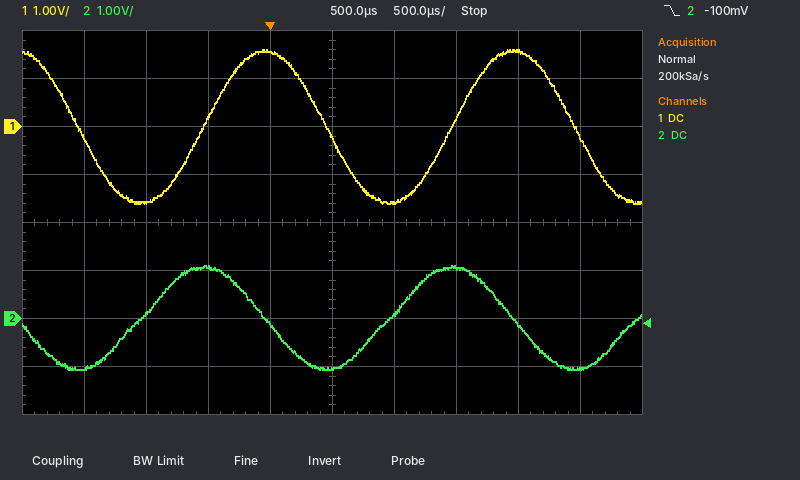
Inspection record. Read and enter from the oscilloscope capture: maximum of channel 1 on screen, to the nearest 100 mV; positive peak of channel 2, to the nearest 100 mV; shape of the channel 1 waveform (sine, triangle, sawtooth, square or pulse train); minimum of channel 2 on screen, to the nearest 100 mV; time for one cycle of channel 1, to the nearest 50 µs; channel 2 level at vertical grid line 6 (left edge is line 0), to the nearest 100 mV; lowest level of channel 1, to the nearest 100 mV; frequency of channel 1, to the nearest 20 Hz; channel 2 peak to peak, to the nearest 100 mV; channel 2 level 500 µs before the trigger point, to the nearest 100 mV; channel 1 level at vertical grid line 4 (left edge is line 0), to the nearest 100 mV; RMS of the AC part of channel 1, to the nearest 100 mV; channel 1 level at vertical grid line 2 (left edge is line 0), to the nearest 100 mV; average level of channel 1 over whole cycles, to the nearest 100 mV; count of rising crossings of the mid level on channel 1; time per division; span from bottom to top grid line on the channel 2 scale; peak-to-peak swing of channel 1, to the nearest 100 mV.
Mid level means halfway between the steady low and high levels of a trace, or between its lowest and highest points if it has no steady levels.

1.6 V
1.1 V
sine
-1.1 V
2.00 ms
100 mV
-1.6 V
500 Hz
2.2 V
1.1 V
1.6 V
1.1 V
-1.6 V
0.0 V
2
500 µs
8 V
3.2 V
